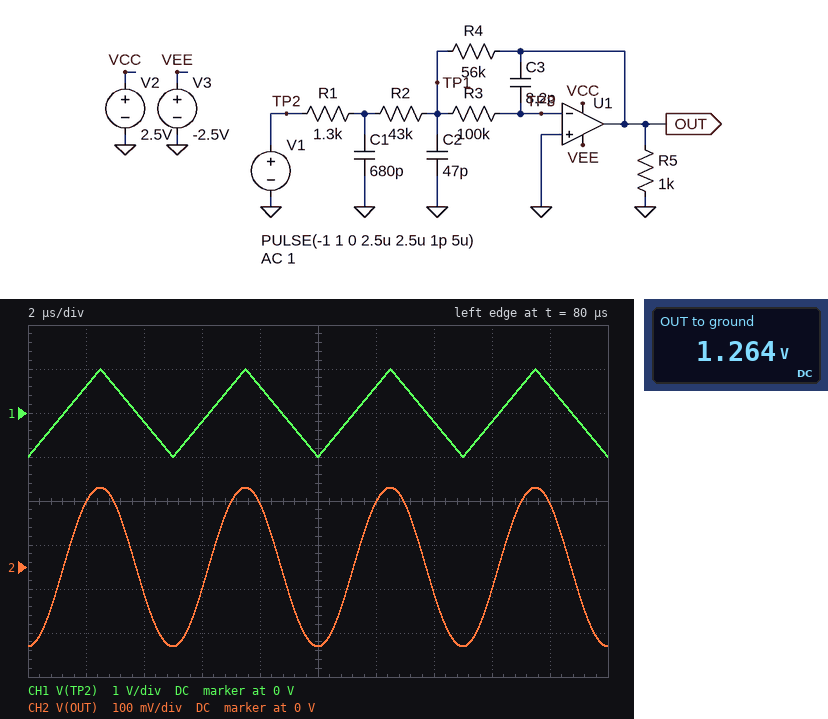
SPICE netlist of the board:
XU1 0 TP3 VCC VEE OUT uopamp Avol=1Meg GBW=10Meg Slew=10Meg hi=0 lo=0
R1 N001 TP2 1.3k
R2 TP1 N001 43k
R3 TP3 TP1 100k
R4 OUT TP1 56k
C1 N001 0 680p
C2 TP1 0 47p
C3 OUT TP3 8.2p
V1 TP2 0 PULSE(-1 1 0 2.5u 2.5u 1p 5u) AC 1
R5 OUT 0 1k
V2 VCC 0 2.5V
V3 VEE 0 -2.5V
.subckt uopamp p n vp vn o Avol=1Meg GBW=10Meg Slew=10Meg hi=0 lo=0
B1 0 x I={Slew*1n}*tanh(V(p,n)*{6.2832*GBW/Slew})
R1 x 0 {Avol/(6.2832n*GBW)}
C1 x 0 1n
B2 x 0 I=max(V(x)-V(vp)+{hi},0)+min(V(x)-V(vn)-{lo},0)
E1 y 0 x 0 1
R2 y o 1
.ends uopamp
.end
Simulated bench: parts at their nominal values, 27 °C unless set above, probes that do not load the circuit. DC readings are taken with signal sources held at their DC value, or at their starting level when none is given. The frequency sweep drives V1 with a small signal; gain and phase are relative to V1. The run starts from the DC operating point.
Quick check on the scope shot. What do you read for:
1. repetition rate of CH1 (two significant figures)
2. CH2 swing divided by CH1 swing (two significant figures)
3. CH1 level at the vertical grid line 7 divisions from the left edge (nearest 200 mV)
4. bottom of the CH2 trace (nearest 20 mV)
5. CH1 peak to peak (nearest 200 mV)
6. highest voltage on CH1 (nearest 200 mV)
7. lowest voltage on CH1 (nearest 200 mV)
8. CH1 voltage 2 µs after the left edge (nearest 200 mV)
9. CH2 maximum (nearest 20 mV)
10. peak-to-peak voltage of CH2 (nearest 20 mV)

200 kHz
0.18
-200 mV
-180 mV
2.0 V
1.0 V
-1.0 V
600 mV
180 mV
360 mV
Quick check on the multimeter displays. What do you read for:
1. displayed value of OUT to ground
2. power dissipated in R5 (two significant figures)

1.264 V
1.6 mW
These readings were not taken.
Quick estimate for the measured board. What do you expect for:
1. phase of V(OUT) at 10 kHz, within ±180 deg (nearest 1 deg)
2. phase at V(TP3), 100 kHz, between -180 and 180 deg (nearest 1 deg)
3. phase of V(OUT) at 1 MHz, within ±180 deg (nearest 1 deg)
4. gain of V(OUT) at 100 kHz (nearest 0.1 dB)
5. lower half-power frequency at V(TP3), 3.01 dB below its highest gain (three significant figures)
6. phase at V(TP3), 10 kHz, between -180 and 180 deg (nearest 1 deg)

168 deg
-24 deg
-75 deg
-2.5 dB
46.1 kHz
78 deg
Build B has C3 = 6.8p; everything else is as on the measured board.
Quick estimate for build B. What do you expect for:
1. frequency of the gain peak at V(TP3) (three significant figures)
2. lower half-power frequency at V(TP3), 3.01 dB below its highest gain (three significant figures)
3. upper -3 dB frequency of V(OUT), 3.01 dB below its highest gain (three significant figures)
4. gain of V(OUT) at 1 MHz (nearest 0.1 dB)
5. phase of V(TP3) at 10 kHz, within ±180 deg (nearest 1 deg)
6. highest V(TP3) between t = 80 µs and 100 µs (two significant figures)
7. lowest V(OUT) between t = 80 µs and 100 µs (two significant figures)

103 kHz
53.0 kHz
99.3 kHz
-50.0 dB
80 deg
4.5 mV
-220 mV
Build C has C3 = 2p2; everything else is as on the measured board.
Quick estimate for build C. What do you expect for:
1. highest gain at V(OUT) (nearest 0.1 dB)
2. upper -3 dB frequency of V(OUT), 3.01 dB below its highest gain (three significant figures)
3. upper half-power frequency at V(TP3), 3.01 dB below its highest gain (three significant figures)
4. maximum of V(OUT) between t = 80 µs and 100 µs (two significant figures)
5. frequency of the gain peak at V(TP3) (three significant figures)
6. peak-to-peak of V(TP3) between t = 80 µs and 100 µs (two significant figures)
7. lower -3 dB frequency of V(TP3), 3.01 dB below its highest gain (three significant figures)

2.4 dB
215 kHz
260 kHz
850 mV
184 kHz
35 mV
116 kHz
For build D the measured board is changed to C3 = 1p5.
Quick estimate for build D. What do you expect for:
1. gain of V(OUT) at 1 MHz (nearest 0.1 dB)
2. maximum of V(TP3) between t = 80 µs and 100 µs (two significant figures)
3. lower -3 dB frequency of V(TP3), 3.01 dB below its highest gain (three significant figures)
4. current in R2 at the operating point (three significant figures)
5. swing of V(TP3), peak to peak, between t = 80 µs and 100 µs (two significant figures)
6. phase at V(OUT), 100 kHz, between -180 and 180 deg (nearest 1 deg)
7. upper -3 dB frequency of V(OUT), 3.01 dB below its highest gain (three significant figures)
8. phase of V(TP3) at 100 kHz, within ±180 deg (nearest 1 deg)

-37.1 dB
22 mV
149 kHz
22.6 µA
44 mV
132 deg
262 kHz
42 deg
